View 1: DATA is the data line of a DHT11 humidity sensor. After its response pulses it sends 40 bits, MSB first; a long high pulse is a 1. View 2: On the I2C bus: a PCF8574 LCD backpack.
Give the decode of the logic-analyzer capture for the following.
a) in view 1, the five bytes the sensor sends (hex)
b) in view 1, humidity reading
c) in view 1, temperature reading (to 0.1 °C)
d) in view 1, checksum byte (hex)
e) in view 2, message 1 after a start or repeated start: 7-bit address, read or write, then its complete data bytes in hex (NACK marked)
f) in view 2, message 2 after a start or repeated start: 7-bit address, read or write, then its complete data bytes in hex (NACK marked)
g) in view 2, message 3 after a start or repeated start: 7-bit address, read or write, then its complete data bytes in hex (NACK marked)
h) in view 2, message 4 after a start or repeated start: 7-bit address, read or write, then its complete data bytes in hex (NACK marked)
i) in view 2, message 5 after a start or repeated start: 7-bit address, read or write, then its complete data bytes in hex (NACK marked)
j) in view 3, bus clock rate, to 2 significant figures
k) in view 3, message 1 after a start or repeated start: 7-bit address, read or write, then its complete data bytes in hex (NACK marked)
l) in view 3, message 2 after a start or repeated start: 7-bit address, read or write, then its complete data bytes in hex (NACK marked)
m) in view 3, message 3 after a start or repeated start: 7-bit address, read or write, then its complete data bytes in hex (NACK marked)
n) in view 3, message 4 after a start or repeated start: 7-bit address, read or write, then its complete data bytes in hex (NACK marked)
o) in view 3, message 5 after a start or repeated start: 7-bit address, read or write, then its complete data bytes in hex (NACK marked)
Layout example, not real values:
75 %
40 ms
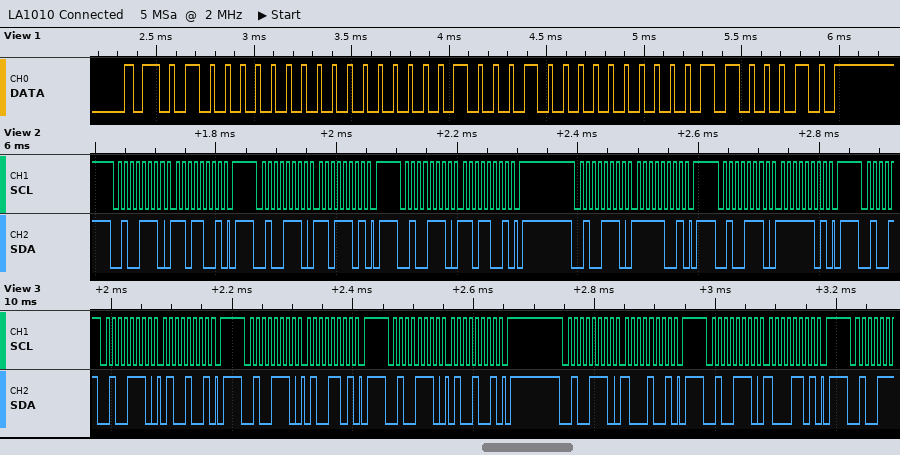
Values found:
40 00 22 00 62
64 %
34.0 °C
0x62
0x27 write: D9
0x27 write: DD
0x27 write: D9
0x27 write: F9
0x27 write: FD
100 kHz
0x27 write: 49
0x27 write: 4D
0x27 write: 49
0x27 write: 89
0x27 write: 8D
